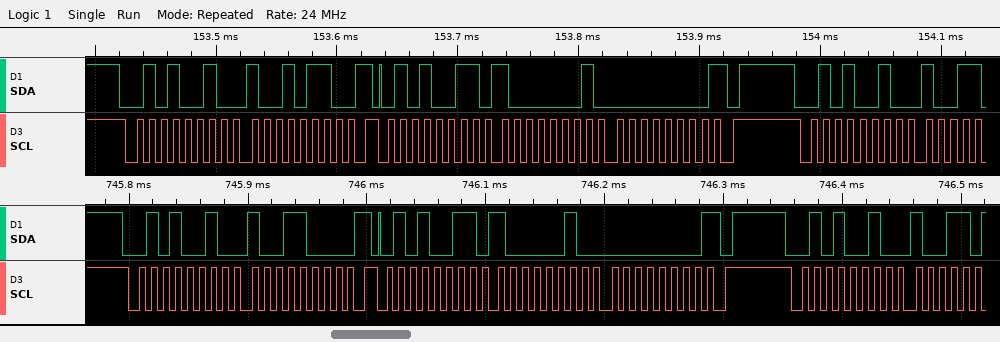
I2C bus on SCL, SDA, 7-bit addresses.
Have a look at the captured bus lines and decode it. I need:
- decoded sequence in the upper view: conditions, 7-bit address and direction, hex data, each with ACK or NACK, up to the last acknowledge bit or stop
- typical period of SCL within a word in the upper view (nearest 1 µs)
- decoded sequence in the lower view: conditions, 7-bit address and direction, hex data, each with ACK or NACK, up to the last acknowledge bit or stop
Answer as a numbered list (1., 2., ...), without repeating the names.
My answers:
1. start, address 29 write ACK, 96 ACK, repeated start, address 29 read ACK, 81 ACK, 00 NACK, stop, start, address 29 write ACK
2. 10 µs
3. start, address 29 write ACK, 98 ACK, repeated start, address 29 read ACK, 82 ACK, 00 NACK, stop, start, address 29 write ACK
